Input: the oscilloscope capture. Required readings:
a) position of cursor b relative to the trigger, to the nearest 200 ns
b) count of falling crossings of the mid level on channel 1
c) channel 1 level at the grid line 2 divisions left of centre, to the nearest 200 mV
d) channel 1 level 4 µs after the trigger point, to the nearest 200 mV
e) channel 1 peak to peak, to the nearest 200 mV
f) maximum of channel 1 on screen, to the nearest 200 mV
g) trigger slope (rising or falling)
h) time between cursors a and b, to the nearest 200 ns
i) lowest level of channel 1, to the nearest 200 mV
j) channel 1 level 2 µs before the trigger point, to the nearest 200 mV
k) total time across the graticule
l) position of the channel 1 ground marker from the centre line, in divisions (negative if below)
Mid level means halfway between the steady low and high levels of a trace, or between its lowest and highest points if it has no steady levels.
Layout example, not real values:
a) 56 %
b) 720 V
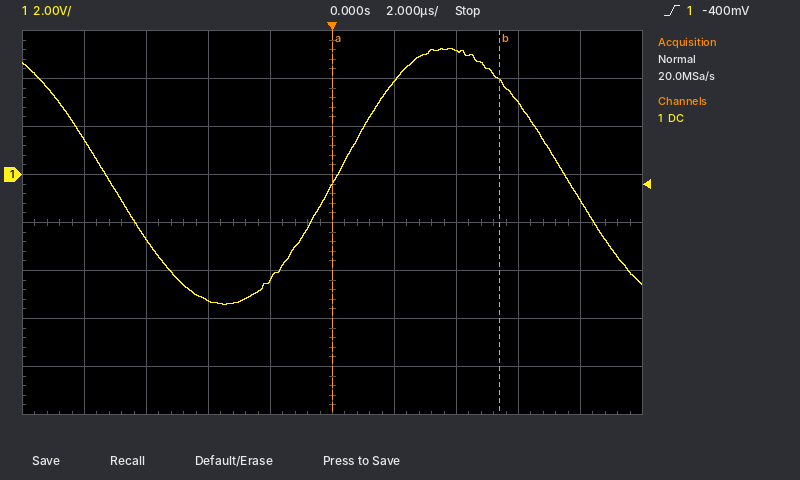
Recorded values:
a) +5.4 µs
b) 2
c) -5.2 V
d) 5.2 V
e) 10.6 V
f) 5.2 V
g) rising
h) 5.4 µs
i) -5.4 V
j) -4.4 V
k) 20 µs
l) +1.0 div
